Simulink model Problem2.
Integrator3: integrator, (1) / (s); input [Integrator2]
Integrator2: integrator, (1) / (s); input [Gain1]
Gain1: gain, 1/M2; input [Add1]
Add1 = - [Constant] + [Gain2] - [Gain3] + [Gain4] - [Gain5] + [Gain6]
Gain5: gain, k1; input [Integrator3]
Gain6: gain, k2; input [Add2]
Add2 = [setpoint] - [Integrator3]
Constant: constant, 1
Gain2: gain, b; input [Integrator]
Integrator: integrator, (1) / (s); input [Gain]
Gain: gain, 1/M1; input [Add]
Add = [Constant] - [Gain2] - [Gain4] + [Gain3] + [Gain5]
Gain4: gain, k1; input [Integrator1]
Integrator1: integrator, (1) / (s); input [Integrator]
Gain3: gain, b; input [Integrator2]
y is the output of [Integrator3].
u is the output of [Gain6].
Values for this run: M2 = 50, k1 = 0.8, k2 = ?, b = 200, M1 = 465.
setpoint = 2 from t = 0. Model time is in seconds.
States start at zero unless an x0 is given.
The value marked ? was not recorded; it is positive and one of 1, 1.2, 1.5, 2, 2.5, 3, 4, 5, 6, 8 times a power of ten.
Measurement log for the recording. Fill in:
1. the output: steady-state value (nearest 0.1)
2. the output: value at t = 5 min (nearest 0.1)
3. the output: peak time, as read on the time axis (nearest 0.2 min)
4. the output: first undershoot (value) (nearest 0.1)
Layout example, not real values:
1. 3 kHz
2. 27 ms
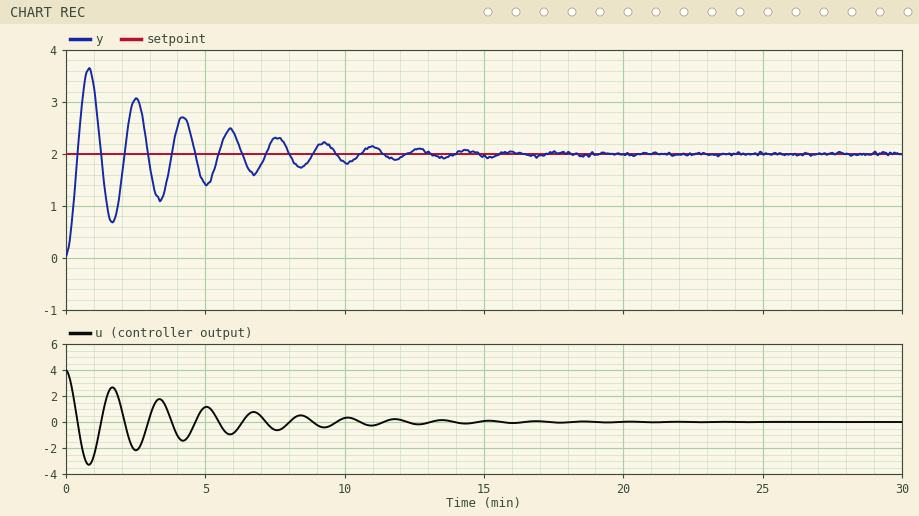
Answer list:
1. 2.0
2. 1.4
3. 0.8 min
4. 0.7
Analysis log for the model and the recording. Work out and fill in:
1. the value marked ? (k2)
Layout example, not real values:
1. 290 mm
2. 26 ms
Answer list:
1. 2
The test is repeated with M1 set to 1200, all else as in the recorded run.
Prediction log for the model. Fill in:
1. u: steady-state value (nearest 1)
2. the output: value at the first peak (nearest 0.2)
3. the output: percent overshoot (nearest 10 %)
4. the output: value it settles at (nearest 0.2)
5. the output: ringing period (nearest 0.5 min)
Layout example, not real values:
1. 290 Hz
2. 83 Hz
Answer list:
1. 0
2. 3.4
3. 70 %
4. 2.0
5. 2.5 min
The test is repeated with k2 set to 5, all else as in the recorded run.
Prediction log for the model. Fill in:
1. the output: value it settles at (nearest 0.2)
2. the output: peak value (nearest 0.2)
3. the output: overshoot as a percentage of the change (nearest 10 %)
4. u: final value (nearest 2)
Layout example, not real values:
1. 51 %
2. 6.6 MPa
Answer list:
1. 2.0
2. 3.4
3. 70 %
4. 0
